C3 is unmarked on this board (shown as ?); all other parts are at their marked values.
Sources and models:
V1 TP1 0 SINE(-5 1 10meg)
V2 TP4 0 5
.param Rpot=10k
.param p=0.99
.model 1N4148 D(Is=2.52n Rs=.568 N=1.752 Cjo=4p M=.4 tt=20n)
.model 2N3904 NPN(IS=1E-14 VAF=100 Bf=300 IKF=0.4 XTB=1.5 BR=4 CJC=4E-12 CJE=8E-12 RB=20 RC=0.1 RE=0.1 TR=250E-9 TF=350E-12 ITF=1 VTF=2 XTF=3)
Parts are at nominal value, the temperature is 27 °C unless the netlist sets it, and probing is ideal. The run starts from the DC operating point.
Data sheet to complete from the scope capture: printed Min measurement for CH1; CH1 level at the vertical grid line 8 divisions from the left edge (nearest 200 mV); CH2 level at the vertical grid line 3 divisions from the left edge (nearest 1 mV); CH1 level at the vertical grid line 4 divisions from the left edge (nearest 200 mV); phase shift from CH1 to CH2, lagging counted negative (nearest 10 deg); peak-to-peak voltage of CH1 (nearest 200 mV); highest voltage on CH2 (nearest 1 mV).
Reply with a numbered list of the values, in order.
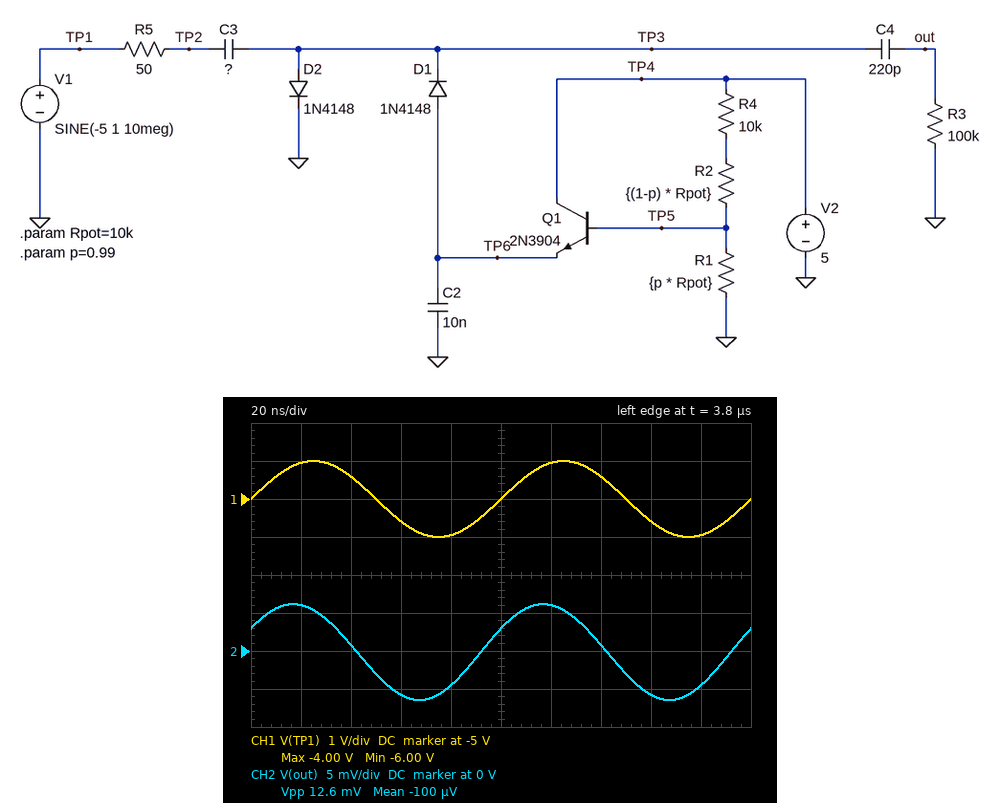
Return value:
1. -6.00 V
2. -5.6 V
3. -6 mV
4. -6.0 V
5. 30 deg
6. 2.0 V
7. 6 mV
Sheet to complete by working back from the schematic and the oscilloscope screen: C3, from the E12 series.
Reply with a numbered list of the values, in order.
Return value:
1. 82 pF
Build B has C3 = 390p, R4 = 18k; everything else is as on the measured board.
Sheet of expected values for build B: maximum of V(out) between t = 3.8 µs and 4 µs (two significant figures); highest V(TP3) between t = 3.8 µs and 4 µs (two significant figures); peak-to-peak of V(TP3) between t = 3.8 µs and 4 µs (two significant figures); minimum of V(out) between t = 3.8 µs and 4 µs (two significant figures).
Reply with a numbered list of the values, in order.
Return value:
1. 130 mV
2. 680 mV
3. 340 mV
4. -210 mV
